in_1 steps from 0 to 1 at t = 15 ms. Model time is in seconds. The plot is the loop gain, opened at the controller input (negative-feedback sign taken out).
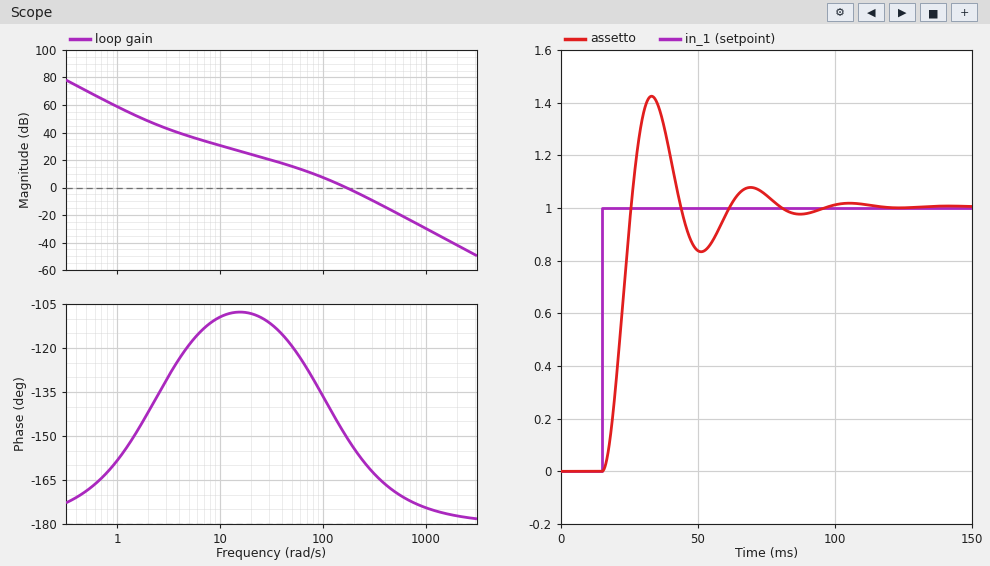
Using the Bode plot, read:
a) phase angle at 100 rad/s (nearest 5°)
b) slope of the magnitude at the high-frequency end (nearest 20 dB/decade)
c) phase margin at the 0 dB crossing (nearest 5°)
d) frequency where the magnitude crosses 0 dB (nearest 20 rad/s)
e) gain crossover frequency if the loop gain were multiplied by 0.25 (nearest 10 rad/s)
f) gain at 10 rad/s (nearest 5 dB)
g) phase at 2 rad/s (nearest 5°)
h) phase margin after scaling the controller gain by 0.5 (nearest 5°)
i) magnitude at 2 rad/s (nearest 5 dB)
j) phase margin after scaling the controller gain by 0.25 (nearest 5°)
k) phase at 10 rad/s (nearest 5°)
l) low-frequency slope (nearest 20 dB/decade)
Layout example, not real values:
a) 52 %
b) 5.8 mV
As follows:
a) -135°
b) -40 dB/decade
c) 30°
d) 160 rad/s
e) 70 rad/s
f) 30 dB
g) -140°
h) 40°
i) 50 dB
j) 55°
k) -110°
l) -40 dB/decade
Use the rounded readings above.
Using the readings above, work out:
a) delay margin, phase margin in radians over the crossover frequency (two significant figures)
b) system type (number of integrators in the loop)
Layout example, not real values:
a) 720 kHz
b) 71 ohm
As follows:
a) 0.0033 s
b) 2
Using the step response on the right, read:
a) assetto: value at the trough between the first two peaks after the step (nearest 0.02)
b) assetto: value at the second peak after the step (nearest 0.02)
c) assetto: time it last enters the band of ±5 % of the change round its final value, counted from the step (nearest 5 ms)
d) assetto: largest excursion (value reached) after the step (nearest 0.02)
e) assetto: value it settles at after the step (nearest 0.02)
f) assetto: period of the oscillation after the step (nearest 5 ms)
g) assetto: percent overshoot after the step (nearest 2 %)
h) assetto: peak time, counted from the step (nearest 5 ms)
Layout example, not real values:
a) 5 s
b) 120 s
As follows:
a) 0.84
b) 1.08
c) 60 ms
d) 1.42
e) 1.00
f) 35 ms
g) 42 %
h) 20 ms
